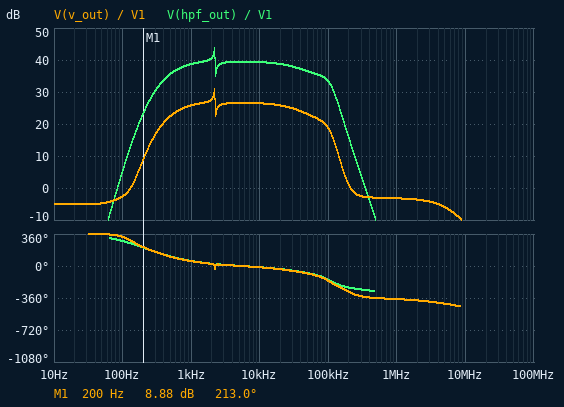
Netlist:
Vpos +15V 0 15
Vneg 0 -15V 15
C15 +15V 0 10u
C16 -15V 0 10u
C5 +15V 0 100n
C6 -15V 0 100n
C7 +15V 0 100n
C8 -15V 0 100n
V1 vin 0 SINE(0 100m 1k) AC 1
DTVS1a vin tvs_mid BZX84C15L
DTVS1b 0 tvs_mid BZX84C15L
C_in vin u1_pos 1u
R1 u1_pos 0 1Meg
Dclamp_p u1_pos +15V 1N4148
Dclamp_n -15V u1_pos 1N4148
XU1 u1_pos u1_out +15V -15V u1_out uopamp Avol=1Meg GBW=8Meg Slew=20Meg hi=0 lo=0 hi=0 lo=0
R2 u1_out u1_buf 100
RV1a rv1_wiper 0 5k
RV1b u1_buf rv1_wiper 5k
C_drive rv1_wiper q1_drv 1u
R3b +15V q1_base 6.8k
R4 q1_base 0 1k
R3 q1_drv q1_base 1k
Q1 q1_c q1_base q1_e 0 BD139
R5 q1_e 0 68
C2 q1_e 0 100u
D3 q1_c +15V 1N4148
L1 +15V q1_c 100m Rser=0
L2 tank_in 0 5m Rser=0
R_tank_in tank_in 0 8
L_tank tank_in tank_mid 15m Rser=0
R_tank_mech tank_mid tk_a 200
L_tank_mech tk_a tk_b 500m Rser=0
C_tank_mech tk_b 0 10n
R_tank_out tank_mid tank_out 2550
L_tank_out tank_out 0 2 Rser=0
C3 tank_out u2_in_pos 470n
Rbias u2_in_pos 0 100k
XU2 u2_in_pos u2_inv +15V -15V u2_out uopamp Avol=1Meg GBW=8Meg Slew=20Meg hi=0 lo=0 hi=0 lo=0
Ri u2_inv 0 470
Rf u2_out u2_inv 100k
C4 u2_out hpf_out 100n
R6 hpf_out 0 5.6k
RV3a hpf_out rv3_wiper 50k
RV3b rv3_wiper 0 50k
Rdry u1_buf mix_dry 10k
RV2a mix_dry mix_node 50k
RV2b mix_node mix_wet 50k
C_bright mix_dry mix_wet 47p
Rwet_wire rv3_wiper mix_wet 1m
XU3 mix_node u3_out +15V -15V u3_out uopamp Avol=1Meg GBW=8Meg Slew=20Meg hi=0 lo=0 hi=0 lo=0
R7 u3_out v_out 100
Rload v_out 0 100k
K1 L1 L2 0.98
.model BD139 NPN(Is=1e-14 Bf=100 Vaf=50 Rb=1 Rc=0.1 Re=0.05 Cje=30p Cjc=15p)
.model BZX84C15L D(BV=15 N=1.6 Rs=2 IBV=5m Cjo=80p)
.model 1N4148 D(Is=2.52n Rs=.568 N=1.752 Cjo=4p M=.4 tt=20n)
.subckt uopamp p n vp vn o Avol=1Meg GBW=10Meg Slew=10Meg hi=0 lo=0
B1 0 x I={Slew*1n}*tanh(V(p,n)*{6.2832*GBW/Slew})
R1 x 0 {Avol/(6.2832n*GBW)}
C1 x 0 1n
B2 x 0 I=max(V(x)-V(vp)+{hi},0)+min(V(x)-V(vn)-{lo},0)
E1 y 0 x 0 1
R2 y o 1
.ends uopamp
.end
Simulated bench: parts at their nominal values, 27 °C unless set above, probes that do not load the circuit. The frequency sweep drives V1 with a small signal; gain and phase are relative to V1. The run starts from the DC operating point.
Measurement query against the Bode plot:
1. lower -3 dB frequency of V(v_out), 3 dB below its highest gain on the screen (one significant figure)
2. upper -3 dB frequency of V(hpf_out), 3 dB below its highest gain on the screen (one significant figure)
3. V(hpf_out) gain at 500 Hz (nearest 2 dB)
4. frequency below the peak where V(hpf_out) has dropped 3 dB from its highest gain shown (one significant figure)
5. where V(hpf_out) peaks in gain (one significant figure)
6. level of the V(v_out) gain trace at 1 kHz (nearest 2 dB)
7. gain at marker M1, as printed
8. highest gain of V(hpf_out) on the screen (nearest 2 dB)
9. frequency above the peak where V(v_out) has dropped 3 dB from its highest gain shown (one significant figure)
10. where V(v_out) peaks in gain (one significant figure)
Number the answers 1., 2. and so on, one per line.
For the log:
1. 2 kHz
2. 2 kHz
3. 36 dB
4. 2 kHz
5. 2 kHz
6. 26 dB
7. 8.88 dB
8. 44 dB
9. 2 kHz
10. 2 kHz
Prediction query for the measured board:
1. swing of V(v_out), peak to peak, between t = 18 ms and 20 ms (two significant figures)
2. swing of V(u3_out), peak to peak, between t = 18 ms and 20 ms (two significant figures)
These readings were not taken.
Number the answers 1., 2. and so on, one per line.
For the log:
1. 3.9 V
2. 3.9 V
